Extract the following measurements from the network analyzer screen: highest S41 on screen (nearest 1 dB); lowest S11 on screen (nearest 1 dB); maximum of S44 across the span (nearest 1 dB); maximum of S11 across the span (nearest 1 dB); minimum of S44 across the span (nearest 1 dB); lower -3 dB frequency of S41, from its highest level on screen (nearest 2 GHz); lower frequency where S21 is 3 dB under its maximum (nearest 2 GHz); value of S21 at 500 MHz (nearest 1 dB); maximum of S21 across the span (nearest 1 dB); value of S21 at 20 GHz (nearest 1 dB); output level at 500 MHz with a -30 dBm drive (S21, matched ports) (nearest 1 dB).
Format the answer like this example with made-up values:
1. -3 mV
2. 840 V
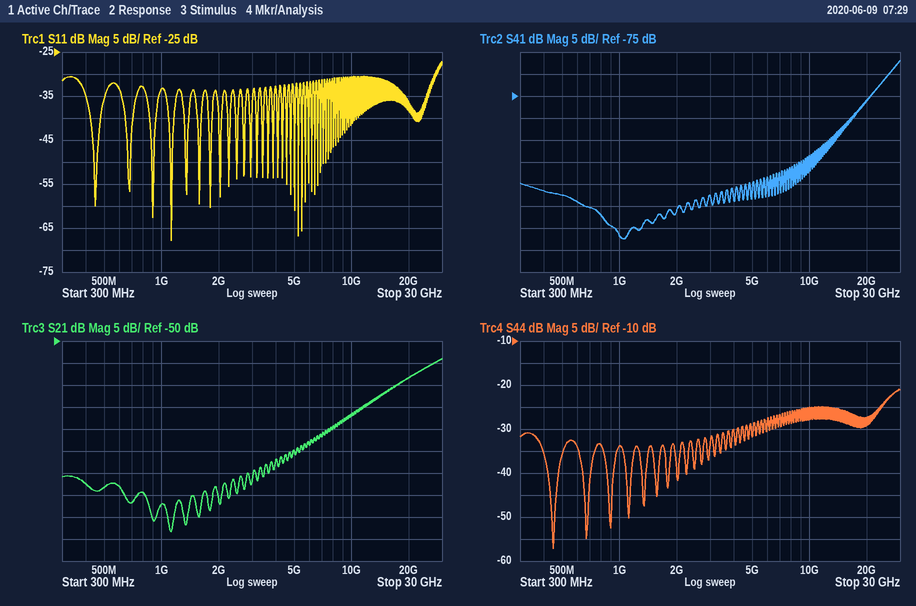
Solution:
1. -67 dB
2. -68 dB
3. -21 dB
4. -27 dB
5. -57 dB
6. 26 GHz
7. 22 GHz
8. -83 dB
9. -54 dB
10. -58 dB
11. -113 dBm
